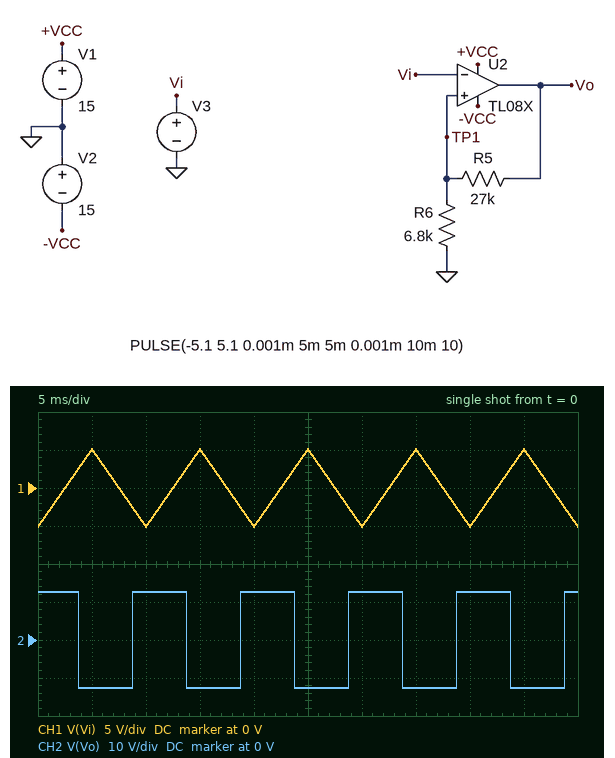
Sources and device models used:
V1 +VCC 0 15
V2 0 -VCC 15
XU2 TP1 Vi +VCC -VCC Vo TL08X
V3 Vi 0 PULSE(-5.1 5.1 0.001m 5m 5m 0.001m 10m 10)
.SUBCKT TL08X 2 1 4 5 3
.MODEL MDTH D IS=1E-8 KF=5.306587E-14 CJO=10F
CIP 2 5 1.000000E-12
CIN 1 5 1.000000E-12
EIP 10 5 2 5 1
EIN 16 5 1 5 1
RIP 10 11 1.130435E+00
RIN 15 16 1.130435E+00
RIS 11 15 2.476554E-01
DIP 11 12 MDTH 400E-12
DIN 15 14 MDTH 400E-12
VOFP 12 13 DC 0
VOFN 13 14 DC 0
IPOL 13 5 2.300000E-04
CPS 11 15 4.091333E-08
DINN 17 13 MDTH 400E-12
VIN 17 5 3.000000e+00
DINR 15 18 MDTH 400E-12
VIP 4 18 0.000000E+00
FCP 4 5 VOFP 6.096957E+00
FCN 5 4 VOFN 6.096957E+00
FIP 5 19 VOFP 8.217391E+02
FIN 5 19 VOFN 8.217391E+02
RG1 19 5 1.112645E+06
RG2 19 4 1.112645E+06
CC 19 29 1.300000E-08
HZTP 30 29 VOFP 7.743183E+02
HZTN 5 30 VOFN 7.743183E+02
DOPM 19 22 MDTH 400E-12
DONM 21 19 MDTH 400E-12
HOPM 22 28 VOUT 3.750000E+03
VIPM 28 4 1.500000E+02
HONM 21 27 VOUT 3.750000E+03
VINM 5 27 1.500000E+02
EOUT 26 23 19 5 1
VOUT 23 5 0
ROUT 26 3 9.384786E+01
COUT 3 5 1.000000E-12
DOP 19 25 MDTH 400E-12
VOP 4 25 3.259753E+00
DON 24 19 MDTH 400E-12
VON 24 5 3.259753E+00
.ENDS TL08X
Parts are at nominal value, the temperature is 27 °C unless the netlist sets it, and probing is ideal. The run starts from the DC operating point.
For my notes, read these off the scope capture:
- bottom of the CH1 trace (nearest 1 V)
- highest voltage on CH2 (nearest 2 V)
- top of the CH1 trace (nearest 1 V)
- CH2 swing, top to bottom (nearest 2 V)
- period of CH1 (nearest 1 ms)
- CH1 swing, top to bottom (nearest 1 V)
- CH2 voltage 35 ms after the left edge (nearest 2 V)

-5 V
12 V
5 V
26 V
10 ms
10 V
-12 V
